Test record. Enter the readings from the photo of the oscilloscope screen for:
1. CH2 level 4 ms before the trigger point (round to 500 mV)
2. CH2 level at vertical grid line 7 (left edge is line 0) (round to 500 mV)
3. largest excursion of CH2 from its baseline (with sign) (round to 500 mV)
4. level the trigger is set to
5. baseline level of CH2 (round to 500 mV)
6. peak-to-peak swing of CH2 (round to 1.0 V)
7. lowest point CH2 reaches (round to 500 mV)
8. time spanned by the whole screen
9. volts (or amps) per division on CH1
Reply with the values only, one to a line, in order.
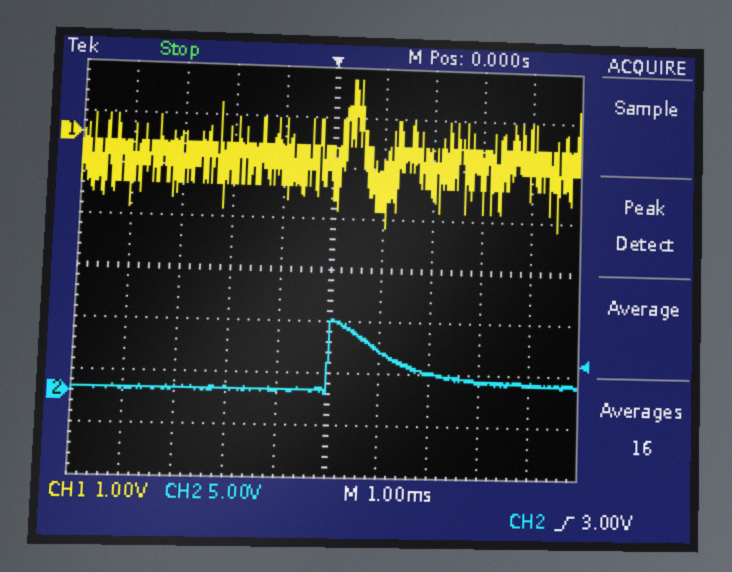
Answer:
500 mV
2.0 V
+7.0 V
3.00 V
500 mV
7.0 V
0.0 V
10 ms
1 V
